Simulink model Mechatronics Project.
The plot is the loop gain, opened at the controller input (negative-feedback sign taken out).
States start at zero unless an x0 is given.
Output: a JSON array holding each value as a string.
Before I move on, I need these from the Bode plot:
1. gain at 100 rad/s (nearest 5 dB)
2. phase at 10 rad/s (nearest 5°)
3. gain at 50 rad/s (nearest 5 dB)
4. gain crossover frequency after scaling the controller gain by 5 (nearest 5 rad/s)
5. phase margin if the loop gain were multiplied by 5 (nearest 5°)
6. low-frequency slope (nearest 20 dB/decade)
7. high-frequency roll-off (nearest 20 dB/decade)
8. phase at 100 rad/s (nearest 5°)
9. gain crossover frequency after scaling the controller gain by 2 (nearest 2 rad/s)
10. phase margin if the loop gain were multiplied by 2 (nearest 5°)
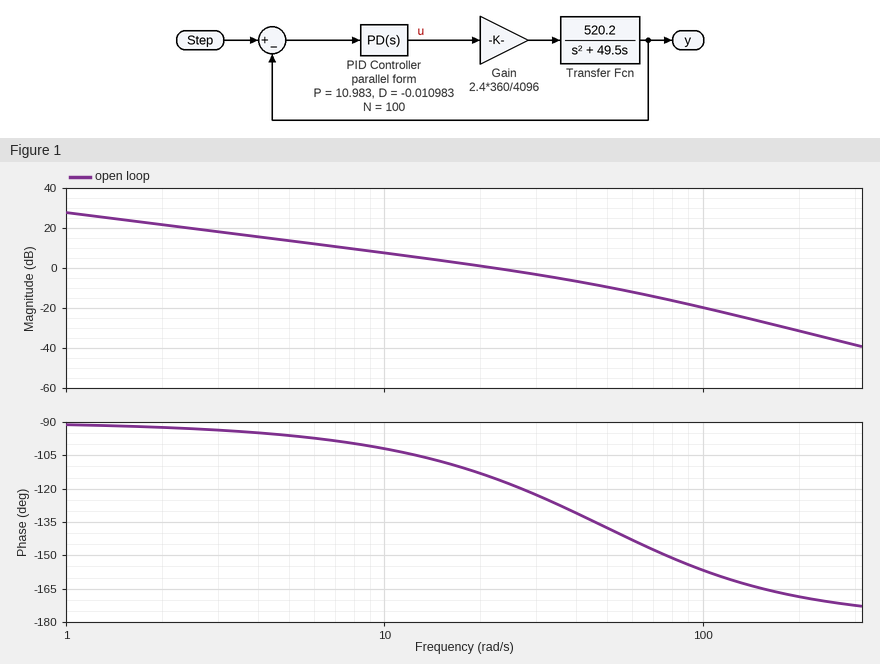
["-20 dB", "-100°", "-10 dB", "70 rad/s", "35°", "-20 dB/decade", "-40 dB/decade", "-155°", "38 rad/s", "50°"]
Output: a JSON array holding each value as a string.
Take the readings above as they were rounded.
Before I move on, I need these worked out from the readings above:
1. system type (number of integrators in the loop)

["1"]
